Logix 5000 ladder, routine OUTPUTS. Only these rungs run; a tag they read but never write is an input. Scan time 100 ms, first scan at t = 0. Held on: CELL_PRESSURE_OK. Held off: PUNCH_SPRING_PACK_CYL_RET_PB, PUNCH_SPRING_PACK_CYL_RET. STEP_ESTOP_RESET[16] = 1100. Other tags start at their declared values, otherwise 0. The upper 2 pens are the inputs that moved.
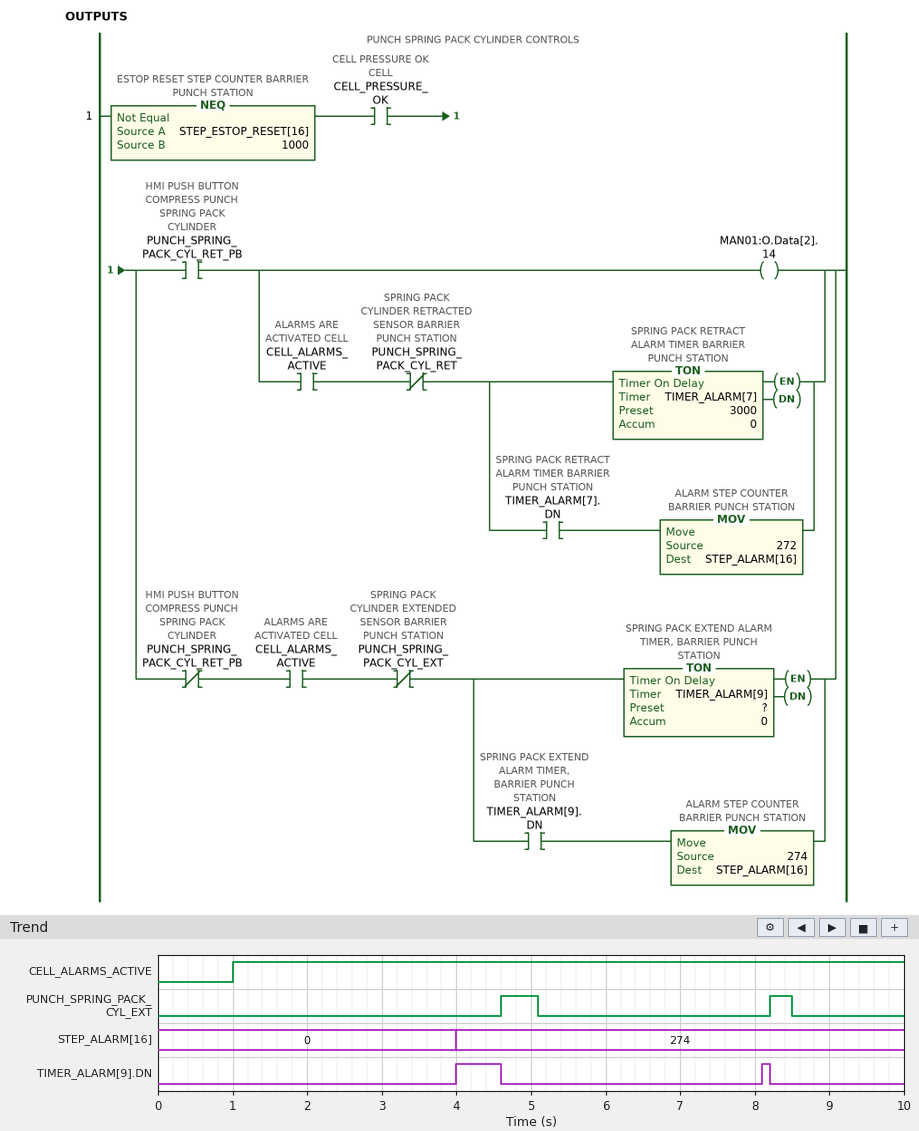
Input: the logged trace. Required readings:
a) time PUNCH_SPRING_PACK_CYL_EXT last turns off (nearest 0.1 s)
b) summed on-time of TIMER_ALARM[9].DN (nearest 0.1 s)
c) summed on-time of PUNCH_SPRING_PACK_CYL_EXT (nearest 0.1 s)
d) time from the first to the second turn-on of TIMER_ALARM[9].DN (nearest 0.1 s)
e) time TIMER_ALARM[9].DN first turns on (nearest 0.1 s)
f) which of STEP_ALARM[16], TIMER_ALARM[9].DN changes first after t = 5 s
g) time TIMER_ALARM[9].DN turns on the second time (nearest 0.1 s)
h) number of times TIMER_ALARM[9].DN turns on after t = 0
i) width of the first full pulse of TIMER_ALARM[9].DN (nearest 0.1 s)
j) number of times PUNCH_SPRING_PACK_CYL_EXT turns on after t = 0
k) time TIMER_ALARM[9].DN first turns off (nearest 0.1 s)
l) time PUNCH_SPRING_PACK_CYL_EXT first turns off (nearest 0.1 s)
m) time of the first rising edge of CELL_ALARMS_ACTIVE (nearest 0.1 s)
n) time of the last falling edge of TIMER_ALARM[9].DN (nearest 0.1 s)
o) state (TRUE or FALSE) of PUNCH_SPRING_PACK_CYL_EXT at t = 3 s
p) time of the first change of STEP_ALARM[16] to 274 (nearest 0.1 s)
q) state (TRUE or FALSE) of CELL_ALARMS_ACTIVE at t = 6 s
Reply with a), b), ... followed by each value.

a) 8.5 s
b) 0.7 s
c) 0.8 s
d) 4.1 s
e) 4.0 s
f) TIMER_ALARM[9].DN
g) 8.1 s
h) 2
i) 0.6 s
j) 2
k) 4.6 s
l) 5.1 s
m) 1.0 s
n) 8.2 s
o) FALSE
p) 4.0 s
q) TRUE
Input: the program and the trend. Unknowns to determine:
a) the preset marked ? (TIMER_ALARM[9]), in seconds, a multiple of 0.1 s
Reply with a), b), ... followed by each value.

a) 3.0 s
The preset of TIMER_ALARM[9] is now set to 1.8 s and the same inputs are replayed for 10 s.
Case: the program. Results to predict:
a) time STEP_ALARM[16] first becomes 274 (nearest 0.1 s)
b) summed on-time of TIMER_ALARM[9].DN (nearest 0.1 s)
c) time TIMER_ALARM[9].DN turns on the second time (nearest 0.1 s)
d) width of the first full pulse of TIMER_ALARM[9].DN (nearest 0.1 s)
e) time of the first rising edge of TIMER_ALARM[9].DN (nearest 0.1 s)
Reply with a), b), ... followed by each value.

a) 2.8 s
b) 3.1 s
c) 6.9 s
d) 1.8 s
e) 2.8 s
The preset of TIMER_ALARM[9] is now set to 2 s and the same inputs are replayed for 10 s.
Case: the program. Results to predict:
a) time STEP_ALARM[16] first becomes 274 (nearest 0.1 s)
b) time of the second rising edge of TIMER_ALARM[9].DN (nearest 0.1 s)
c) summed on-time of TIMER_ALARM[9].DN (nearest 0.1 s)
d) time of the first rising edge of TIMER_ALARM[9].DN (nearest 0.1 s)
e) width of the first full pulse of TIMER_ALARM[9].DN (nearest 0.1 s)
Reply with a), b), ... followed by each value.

a) 3.0 s
b) 7.1 s
c) 2.7 s
d) 3.0 s
e) 1.6 s
